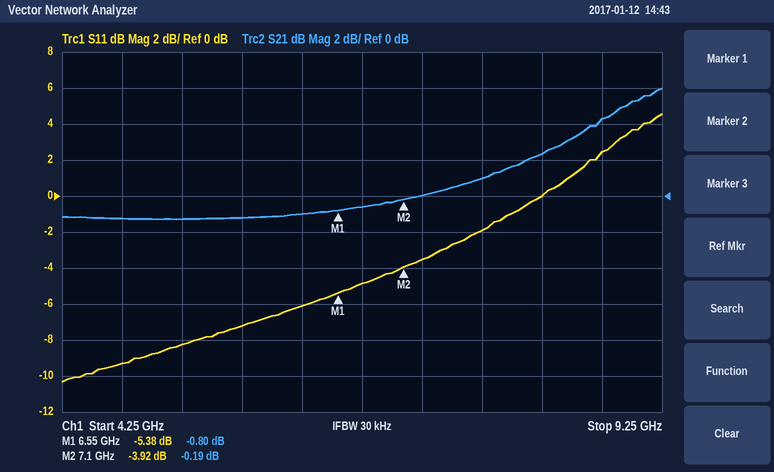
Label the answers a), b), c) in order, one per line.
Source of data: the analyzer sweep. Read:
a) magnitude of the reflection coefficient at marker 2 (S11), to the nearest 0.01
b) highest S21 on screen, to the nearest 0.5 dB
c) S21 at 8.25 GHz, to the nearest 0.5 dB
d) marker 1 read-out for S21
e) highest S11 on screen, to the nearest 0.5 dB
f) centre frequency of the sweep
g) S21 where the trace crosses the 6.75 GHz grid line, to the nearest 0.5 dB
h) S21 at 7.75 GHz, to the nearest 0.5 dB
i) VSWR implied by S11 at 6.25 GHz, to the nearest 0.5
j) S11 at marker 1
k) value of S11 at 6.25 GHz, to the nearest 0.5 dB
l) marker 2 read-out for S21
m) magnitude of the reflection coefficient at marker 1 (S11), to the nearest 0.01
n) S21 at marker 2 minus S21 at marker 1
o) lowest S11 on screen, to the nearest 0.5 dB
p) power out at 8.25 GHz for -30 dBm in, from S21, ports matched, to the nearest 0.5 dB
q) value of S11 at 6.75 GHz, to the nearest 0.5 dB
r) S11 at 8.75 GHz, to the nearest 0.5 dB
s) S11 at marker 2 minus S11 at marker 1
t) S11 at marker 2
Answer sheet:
a) 0.64
b) 6.0 dB
c) 2.5 dB
d) -0.80 dB
e) 4.5 dB
f) 6.75 GHz
g) -0.5 dB
h) 1.0 dB
i) 3.0
j) -5.38 dB
k) -6.0 dB
l) -0.19 dB
m) 0.54
n) 0.61 dB
o) -10.5 dB
p) -27.5 dBm
q) -5.0 dB
r) 2.5 dB
s) 1.46 dB
t) -3.92 dB
